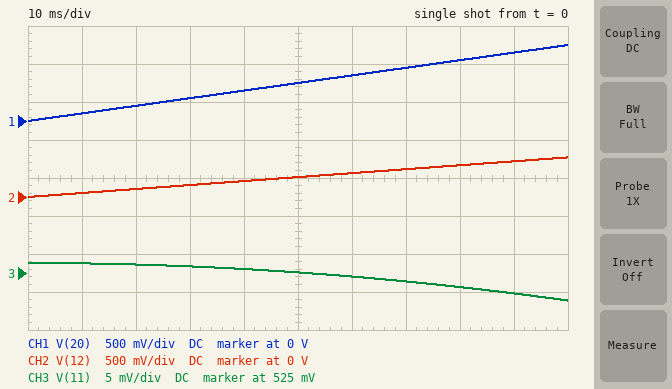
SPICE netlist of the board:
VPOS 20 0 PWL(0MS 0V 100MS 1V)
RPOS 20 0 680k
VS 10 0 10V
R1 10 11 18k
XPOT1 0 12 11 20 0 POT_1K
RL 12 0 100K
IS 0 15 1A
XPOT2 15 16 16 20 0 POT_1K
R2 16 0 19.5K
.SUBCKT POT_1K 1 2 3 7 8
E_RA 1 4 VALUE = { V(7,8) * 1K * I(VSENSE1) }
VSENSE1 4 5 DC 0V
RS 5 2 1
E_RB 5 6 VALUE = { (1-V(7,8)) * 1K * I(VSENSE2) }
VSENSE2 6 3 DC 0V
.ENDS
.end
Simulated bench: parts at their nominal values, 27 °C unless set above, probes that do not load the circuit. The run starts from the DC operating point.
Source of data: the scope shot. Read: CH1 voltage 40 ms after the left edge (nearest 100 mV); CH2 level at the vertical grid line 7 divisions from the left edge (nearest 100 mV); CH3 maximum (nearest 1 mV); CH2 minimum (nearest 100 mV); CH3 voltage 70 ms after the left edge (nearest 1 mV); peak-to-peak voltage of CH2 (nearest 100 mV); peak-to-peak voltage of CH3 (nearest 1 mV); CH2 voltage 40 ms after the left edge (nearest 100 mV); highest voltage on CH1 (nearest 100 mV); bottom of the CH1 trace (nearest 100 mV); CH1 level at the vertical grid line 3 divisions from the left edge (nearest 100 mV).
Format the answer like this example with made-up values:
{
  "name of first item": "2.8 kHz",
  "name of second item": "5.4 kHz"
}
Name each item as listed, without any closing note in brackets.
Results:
{
  "CH1 voltage 40 ms after the left edge": "400 mV",
  "CH2 level at the vertical grid line 7 divisions from the left edge": "400 mV",
  "CH3 maximum": "526 mV",
  "CH2 minimum": "0 V",
  "CH3 voltage 70 ms after the left edge": "524 mV",
  "peak-to-peak voltage of CH2": "500 mV",
  "peak-to-peak voltage of CH3": "5 mV",
  "CH2 voltage 40 ms after the left edge": "200 mV",
  "highest voltage on CH1": "1.0 V",
  "bottom of the CH1 trace": "0 V",
  "CH1 level at the vertical grid line 3 divisions from the left edge": "300 mV"
}
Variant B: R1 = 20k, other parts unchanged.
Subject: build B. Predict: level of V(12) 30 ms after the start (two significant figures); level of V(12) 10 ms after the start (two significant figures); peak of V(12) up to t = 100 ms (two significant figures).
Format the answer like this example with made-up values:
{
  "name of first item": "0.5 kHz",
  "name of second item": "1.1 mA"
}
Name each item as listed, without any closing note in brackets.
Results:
{
  "level of V(12) 30 ms after the start": "140 mV",
  "level of V(12) 10 ms after the start": "48 mV",
  "peak of V(12) up to t = 100 ms": "470 mV"
}
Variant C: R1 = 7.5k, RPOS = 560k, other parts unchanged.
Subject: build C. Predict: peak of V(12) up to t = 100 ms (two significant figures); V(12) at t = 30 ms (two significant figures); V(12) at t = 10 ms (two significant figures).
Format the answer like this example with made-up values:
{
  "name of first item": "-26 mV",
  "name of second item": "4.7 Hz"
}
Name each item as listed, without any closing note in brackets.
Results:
{
  "peak of V(12) up to t = 100 ms": "1.2 V",
  "V(12) at t = 30 ms": "350 mV",
  "V(12) at t = 10 ms": "120 mV"
}
